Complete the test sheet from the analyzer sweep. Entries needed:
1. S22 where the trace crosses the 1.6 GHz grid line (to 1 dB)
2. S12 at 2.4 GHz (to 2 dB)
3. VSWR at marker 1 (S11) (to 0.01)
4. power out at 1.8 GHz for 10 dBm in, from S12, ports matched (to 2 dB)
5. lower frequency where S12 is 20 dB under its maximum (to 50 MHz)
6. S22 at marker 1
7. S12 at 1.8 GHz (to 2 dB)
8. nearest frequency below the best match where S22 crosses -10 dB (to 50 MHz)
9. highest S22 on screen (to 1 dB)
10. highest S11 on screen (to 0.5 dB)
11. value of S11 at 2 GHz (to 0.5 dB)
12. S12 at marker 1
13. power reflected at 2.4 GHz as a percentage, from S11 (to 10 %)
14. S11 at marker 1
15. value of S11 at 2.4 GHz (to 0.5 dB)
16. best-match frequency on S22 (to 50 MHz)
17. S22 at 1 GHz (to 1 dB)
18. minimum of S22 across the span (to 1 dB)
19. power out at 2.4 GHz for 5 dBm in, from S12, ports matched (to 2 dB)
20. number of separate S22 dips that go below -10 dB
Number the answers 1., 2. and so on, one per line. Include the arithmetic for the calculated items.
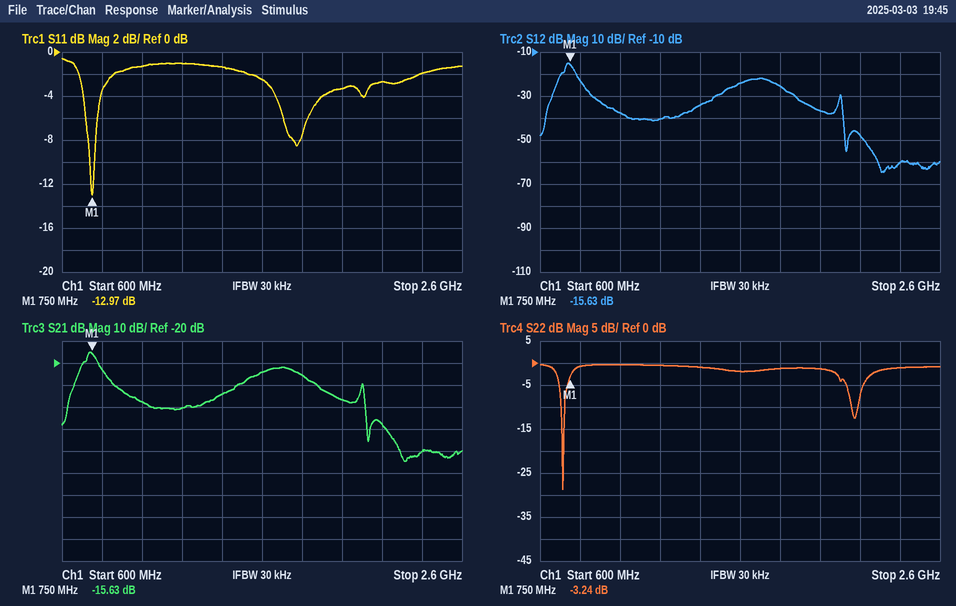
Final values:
1. -2 dB
2. -60 dB
3. (1 + 0.2246)/(1 − 0.2246) ≈ 1.58
4. 10 dBm + (-26 dB) = -16 dBm
5. 650 MHz
6. -3.24 dB
7. -26 dB
8. 700 MHz
9. 0 dB
10. -0.5 dB
11. -3.5 dB
12. -15.63 dB
13. 10^(-2/10) ≈ 63.1 %, so 60 % to the nearest 10 %
14. -12.97 dB
15. -2.0 dB
16. 700 MHz
17. 0 dB
18. -29 dB
19. 5 dBm + (-60 dB) = -56 dBm
20. 2
